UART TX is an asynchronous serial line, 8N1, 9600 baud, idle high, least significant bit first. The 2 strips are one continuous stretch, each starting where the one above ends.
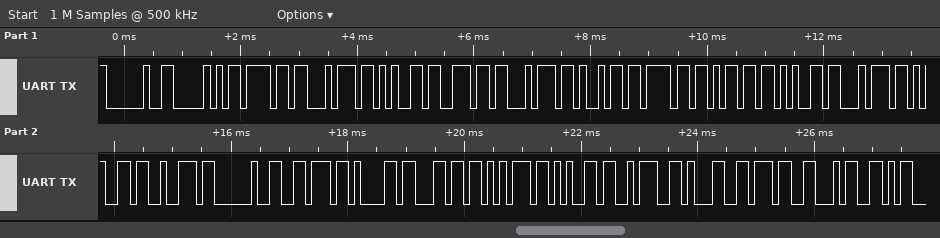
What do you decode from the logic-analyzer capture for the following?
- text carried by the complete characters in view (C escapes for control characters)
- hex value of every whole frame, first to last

" Potentiometer value:174"
20 50 6F 74 65 6E 74 69 6F 6D 65 74 65 72 20 76 61 6C 75 65 3A 31 37 34
